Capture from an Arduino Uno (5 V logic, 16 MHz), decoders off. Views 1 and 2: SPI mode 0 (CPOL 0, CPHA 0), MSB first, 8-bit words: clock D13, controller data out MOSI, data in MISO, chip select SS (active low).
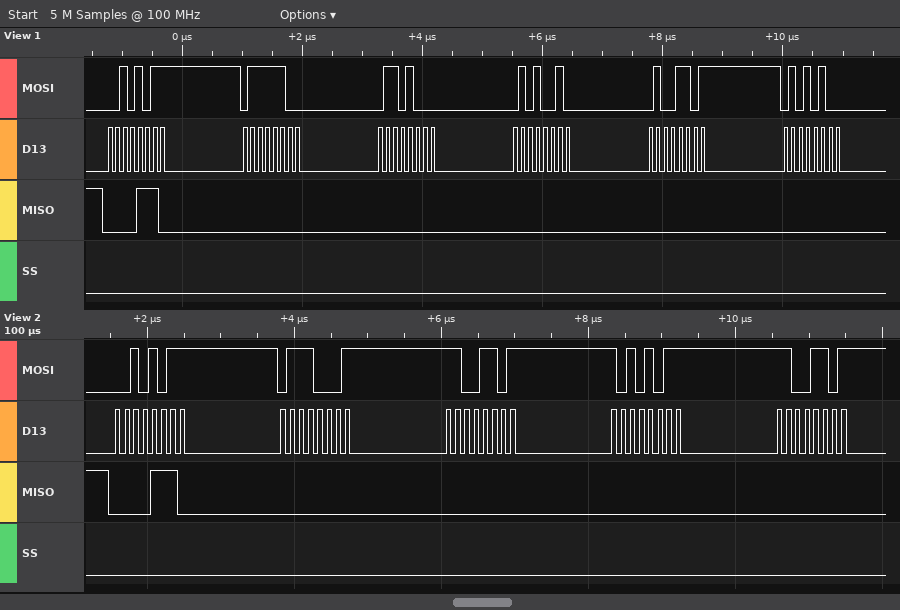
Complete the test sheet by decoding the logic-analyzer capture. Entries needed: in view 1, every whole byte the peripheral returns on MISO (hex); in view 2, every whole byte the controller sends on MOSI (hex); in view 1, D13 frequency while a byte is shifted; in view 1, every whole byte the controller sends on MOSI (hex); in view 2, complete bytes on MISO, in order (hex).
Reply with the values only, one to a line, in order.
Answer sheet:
0E 00 00 00 00 00
2B 71 CD AB CD
8 MHz
2B 7C 68 52 4D 54
0E 00 00 00 00
